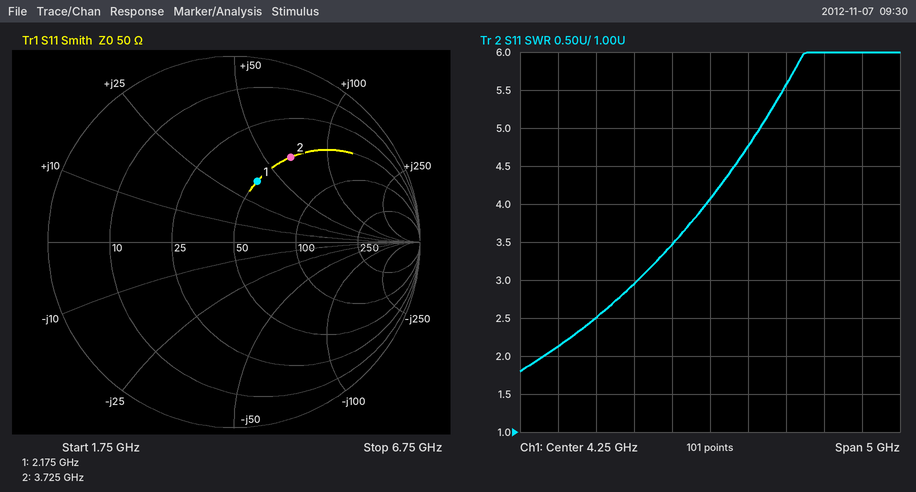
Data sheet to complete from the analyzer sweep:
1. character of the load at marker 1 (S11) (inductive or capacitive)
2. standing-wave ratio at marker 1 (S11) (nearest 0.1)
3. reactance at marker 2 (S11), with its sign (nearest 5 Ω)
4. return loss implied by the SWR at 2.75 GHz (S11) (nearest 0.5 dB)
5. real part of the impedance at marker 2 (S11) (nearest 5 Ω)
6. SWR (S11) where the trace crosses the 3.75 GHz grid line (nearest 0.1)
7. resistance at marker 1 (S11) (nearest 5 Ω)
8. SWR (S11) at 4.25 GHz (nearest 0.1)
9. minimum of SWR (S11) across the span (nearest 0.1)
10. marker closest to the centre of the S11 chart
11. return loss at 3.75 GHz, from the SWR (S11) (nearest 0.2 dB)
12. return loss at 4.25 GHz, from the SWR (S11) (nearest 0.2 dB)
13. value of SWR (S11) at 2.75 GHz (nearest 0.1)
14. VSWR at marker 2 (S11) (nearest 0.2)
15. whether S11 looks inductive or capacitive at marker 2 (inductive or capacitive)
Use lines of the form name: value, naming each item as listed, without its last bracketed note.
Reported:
character of the load at marker 1 (S11): inductive
standing-wave ratio at marker 1 (S11): 2.1
reactance at marker 2 (S11), with its sign: +65 Ω
return loss implied by the SWR at 2.75 GHz (S11): 7.5 dB
real part of the impedance at marker 2 (S11): 50 Ω
SWR (S11) where the trace crosses the 3.75 GHz grid line: 3.5
resistance at marker 1 (S11): 50 Ω
SWR (S11) at 4.25 GHz: 4.1
minimum of SWR (S11) across the span: 1.8
marker closest to the centre of the S11 chart: marker 1
return loss at 3.75 GHz, from the SWR (S11): 5.2 dB
return loss at 4.25 GHz, from the SWR (S11): 4.4 dB
value of SWR (S11) at 2.75 GHz: 2.5
VSWR at marker 2 (S11): 3.4
whether S11 looks inductive or capacitive at marker 2: inductive
